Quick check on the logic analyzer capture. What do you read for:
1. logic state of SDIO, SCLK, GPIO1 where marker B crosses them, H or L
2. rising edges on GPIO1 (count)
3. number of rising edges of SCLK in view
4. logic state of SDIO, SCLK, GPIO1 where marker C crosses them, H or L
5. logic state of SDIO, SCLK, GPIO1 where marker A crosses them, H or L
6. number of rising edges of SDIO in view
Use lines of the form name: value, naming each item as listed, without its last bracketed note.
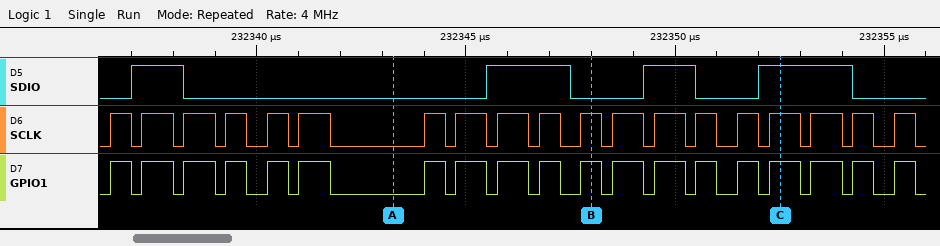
logic state of SDIO, SCLK, GPIO1 where marker B crosses them, H or L: SDIO=L, SCLK=H, GPIO1=H
rising edges on GPIO1: 19
number of rising edges of SCLK in view: 19
logic state of SDIO, SCLK, GPIO1 where marker C crosses them, H or L: SDIO=H, SCLK=H, GPIO1=H
logic state of SDIO, SCLK, GPIO1 where marker A crosses them, H or L: SDIO=L, SCLK=L, GPIO1=L
number of rising edges of SDIO in view: 4
